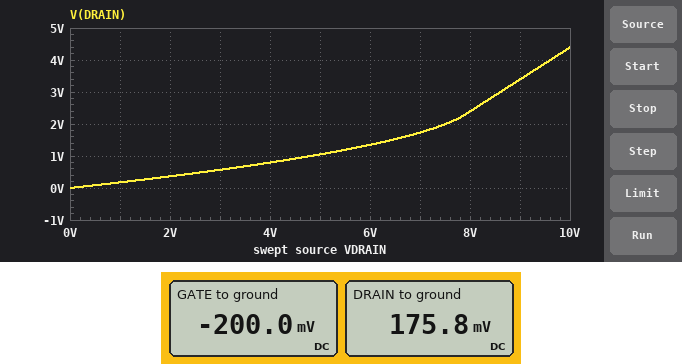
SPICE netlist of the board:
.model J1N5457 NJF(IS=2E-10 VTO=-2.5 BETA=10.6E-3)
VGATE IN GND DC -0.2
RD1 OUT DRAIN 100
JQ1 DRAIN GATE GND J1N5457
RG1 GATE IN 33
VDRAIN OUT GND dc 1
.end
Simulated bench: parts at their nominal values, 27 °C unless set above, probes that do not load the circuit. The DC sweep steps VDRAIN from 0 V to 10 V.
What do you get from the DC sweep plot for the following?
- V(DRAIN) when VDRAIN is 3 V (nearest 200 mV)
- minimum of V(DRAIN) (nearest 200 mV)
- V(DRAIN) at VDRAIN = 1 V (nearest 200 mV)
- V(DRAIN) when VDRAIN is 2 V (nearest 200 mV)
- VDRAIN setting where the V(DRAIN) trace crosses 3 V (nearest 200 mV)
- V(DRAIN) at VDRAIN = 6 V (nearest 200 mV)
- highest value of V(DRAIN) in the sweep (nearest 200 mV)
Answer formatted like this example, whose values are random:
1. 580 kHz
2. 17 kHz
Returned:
1. 600 mV
2. 0 V
3. 200 mV
4. 400 mV
5. 8.6 V
6. 1.4 V
7. 4.4 V
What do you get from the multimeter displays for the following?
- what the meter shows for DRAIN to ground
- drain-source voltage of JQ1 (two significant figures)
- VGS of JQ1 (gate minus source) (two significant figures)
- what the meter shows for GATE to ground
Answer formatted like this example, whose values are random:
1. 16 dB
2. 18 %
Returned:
1. 175.8 mV
2. 180 mV
3. -200 mV
4. -200.0 mV
